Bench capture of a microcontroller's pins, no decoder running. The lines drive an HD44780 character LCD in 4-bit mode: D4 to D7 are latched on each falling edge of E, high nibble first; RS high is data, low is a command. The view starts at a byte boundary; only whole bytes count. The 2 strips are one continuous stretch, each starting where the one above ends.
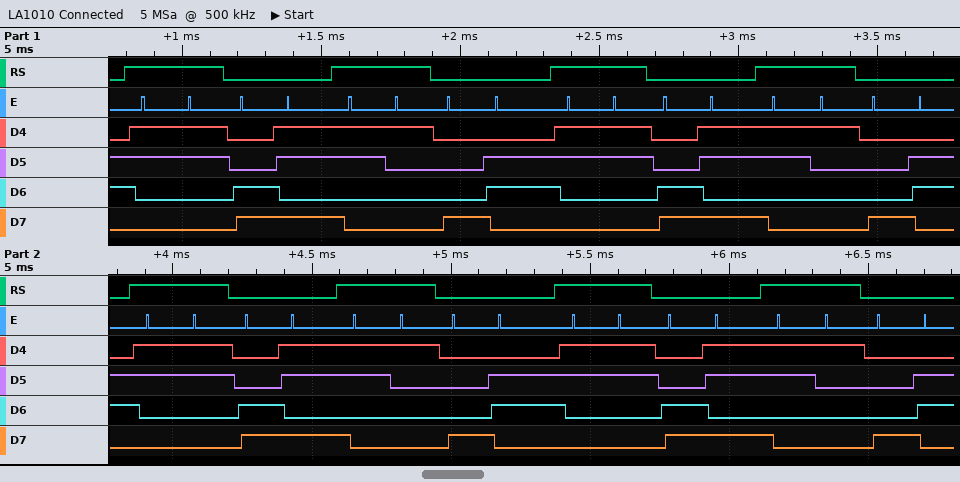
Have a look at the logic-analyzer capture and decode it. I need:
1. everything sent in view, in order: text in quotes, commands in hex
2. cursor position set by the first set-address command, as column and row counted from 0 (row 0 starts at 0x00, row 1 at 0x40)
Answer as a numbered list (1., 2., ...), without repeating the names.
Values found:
1. "3" 0xCB "1" 0x86 "3" 0xCB "1" 0x86 "3" 0xCB "1" 0x86 "3" 0xCB "1" 0x86
2. column 11, row 1
